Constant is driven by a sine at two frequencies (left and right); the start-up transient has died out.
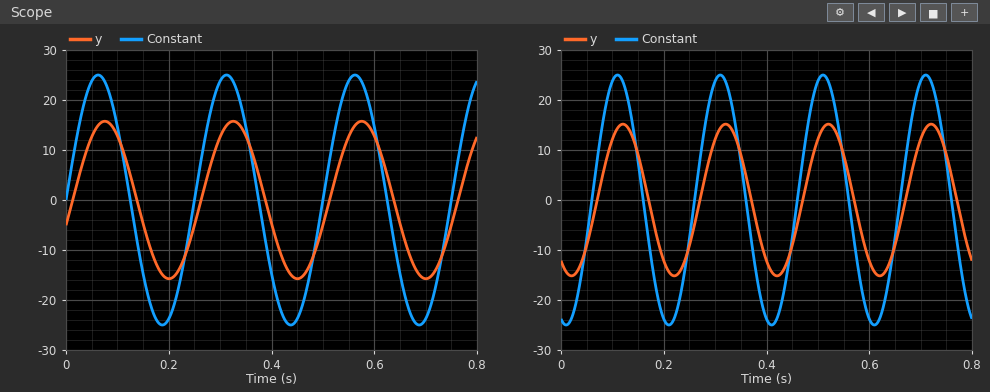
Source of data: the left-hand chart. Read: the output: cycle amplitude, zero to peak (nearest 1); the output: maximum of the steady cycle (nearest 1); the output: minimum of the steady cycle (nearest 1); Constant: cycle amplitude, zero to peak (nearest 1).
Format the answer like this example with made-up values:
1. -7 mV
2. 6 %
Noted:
1. 16
2. 16
3. -16
4. 25
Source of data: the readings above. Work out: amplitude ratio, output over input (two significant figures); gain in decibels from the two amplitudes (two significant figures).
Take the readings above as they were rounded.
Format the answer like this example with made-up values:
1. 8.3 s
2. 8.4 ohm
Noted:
1. 0.64
2. -3.9 dB
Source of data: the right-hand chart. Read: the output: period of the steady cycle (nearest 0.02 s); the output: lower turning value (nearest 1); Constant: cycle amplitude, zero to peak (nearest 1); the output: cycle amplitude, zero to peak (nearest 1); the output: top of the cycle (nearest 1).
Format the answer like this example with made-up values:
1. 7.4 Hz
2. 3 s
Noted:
1. 0.20 s
2. -15
3. 25
4. 15
5. 15
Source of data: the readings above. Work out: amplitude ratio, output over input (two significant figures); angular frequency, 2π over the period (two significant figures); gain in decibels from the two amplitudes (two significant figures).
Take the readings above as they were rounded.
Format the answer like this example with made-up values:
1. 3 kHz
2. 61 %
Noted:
1. 0.60
2. 31 rad/s
3. -4.4 dB
